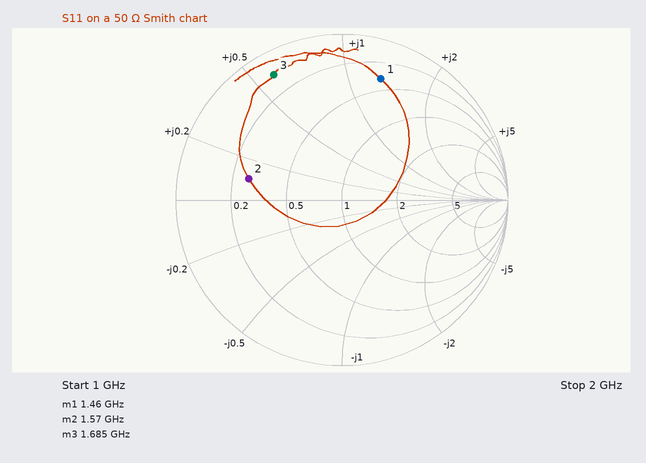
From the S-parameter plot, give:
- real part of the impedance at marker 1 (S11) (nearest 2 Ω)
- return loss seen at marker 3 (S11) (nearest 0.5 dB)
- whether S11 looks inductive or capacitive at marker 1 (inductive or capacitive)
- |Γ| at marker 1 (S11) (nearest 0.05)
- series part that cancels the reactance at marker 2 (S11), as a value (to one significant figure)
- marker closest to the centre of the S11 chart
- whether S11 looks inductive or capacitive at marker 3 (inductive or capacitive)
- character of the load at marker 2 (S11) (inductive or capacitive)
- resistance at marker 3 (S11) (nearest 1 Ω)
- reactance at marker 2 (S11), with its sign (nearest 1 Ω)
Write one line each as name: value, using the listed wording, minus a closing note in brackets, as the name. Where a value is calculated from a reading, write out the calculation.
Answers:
real part of the impedance at marker 1 (S11): 18 Ω
return loss seen at marker 3 (S11): 1.5 dB
whether S11 looks inductive or capacitive at marker 1: inductive
|Γ| at marker 1 (S11): 0.75
series part that cancels the reactance at marker 2 (S11), as a value: C = 1/(2π × 1.57 GHz × 5 Ω) ≈ 20 pF
marker closest to the centre of the S11 chart: marker 2
whether S11 looks inductive or capacitive at marker 3: inductive
character of the load at marker 2 (S11): inductive
resistance at marker 3 (S11): 5 Ω
reactance at marker 2 (S11), with its sign: +5 Ω
